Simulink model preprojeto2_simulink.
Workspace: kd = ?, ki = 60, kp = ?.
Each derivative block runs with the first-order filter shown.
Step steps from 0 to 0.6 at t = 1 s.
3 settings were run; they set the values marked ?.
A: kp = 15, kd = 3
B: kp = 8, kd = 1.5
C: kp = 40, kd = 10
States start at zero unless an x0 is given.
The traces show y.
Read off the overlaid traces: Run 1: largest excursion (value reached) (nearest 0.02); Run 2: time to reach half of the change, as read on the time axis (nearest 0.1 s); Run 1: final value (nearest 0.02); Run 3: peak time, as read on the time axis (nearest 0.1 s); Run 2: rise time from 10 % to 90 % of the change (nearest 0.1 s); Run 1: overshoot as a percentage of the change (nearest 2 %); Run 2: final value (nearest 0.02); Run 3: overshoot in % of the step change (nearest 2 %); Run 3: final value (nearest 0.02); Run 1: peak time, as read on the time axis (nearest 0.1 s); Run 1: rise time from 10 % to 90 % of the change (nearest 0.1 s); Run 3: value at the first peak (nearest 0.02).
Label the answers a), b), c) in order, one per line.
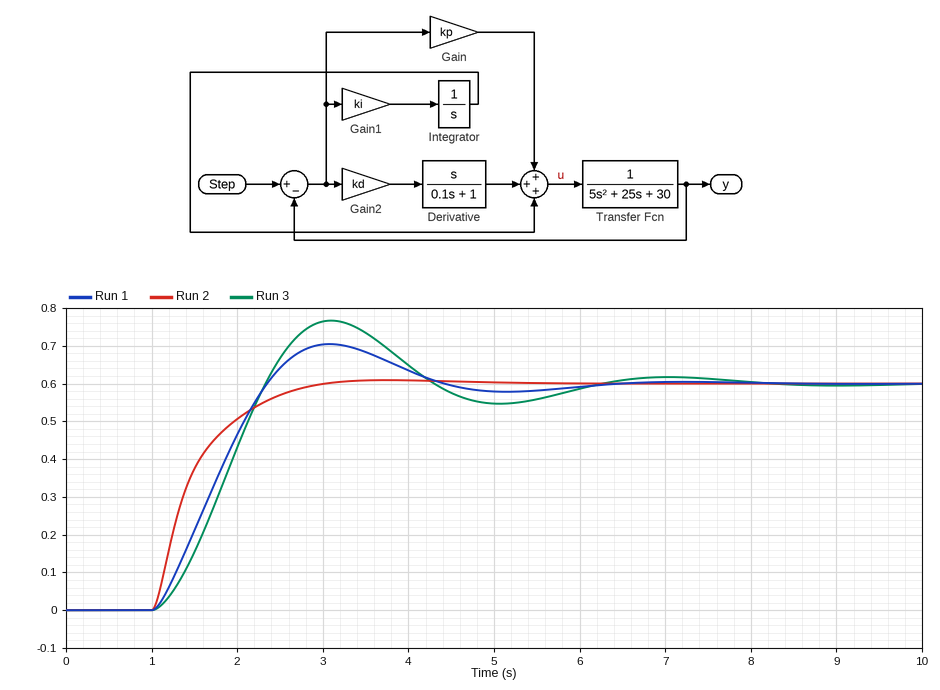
a) 0.70
b) 1.4 s
c) 0.60
d) 3.1 s
e) 1.1 s
f) 18 %
g) 0.60
h) 28 %
i) 0.60
j) 3.1 s
k) 1.0 s
l) 0.76
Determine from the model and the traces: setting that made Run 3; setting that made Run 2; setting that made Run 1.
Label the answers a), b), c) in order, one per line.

a) B
b) C
c) A
